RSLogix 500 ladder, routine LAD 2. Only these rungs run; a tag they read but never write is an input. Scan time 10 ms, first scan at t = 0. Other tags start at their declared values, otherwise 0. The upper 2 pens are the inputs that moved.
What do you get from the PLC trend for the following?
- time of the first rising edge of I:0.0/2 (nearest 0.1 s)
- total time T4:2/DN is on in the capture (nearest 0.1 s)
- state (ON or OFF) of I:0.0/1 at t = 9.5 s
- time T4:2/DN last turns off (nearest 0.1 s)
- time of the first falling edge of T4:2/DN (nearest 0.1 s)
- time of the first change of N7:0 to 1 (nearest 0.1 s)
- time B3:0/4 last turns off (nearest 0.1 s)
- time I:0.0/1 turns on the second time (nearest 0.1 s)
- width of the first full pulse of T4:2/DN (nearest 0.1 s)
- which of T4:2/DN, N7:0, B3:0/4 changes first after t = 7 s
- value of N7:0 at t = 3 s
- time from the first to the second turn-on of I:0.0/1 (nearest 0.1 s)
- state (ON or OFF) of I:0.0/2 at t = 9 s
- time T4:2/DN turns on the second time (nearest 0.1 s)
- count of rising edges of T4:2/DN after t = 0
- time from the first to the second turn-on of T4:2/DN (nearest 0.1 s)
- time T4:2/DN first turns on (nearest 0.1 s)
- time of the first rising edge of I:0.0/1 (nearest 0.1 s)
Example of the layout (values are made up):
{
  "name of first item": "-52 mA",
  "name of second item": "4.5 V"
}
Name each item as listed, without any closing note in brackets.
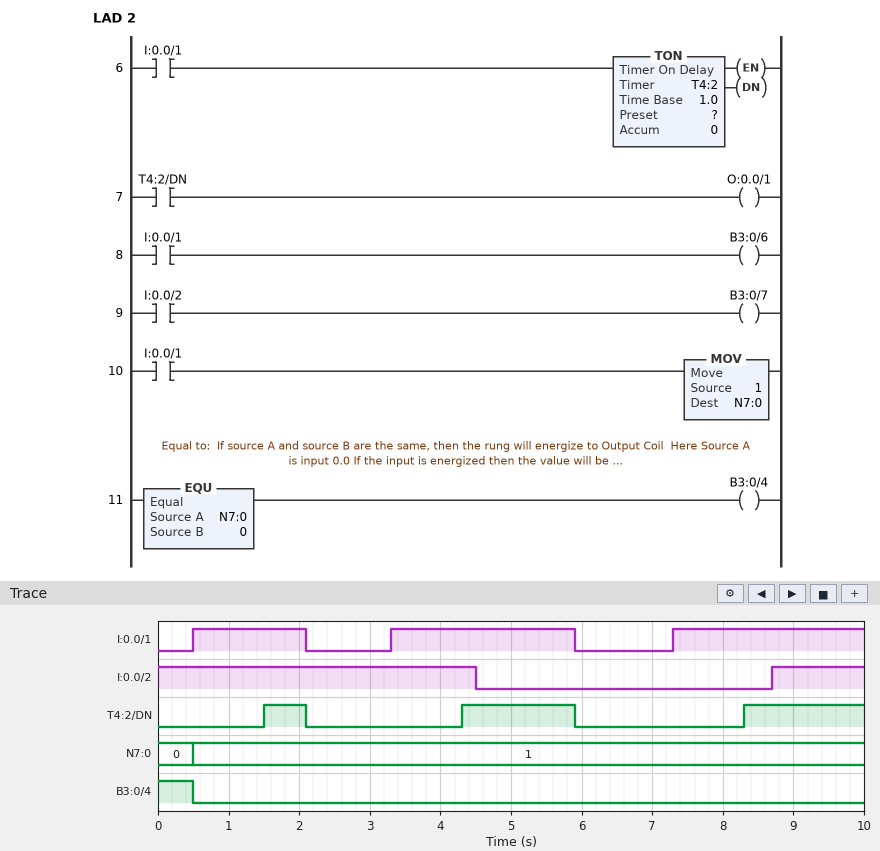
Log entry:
{
  "time of the first rising edge of I:0.0/2": "8.7 s",
  "total time T4:2/DN is on in the capture": "3.9 s",
  "state (ON or OFF) of I:0.0/1 at t = 9.5 s": "ON",
  "time T4:2/DN last turns off": "5.9 s",
  "time of the first falling edge of T4:2/DN": "2.1 s",
  "time of the first change of N7:0 to 1": "0.5 s",
  "time B3:0/4 last turns off": "0.5 s",
  "time I:0.0/1 turns on the second time": "3.3 s",
  "width of the first full pulse of T4:2/DN": "0.6 s",
  "which of T4:2/DN, N7:0, B3:0/4 changes first after t = 7 s": "T4:2/DN",
  "value of N7:0 at t = 3 s": "1",
  "time from the first to the second turn-on of I:0.0/1": "2.8 s",
  "state (ON or OFF) of I:0.0/2 at t = 9 s": "ON",
  "time T4:2/DN turns on the second time": "4.3 s",
  "count of rising edges of T4:2/DN after t = 0": "3",
  "time from the first to the second turn-on of T4:2/DN": "2.8 s",
  "time T4:2/DN first turns on": "1.5 s",
  "time of the first rising edge of I:0.0/1": "0.5 s"
}
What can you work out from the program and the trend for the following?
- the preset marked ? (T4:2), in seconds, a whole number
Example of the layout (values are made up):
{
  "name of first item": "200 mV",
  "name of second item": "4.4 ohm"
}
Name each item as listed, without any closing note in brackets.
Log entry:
{
  "the preset marked ? (T4:2), in seconds, a whole number": "1 s"
}
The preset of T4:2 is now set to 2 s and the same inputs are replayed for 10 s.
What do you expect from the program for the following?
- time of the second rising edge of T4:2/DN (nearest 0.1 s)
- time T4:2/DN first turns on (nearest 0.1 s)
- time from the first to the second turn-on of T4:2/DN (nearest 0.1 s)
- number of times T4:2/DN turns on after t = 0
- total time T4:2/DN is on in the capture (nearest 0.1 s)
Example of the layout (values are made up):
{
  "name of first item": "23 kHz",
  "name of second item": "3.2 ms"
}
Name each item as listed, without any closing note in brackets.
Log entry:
{
  "time of the second rising edge of T4:2/DN": "9.3 s",
  "time T4:2/DN first turns on": "5.3 s",
  "time from the first to the second turn-on of T4:2/DN": "4.0 s",
  "number of times T4:2/DN turns on after t = 0": "2",
  "total time T4:2/DN is on in the capture": "1.3 s"
}
